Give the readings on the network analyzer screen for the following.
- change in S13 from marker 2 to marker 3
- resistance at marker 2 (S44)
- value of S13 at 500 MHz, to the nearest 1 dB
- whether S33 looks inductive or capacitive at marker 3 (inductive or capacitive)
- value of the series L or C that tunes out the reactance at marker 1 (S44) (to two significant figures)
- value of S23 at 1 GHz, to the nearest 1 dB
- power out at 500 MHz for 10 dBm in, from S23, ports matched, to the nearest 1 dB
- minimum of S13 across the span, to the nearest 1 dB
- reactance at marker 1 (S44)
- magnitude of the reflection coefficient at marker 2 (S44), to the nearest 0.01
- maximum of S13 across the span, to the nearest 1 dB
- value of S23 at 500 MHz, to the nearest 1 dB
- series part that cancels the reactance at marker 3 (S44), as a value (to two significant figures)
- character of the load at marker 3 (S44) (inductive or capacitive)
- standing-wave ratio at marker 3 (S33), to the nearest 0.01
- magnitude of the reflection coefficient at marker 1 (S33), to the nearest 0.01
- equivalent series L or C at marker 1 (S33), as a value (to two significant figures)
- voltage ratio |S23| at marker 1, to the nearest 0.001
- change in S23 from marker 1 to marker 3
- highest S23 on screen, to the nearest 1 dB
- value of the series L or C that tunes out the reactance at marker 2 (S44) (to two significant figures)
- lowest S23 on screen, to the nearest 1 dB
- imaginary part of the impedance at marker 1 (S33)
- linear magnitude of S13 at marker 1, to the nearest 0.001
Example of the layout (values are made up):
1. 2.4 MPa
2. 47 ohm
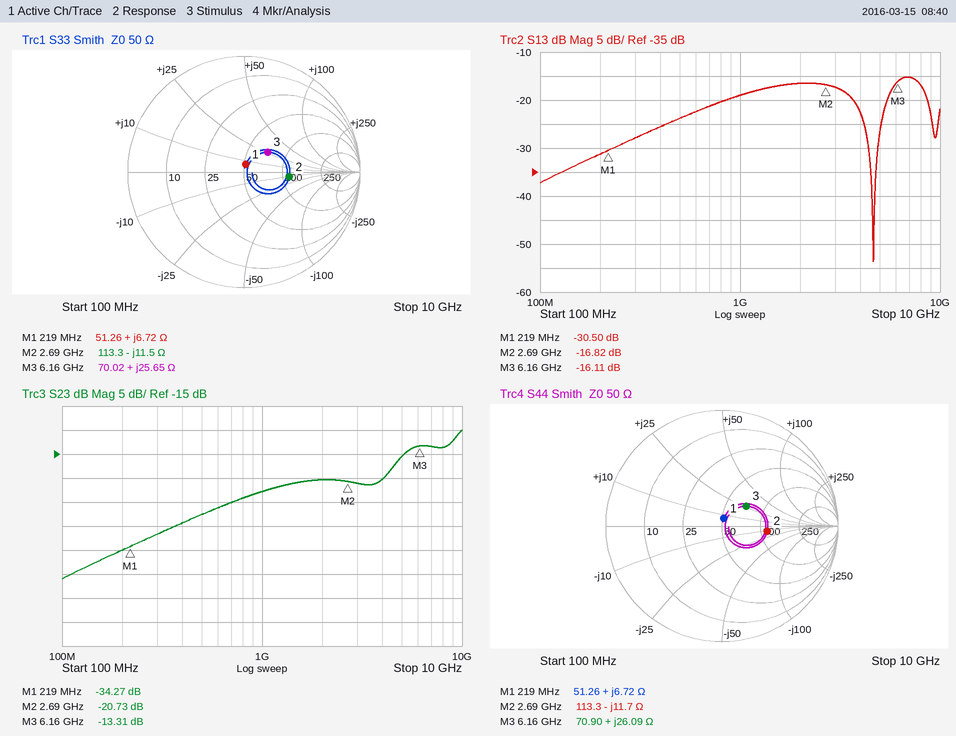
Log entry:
1. 0.71 dB
2. 113.3 Ω
3. -24 dB
4. inductive
5. 110 pF
6. -23 dB
7. -18 dBm
8. -54 dB
9. +6.72 Ω
10. 0.39
11. -15 dB
12. -28 dB
13. 990 fF
14. inductive
15. 1.72
16. 0.07
17. 4.9 nH
18. 0.019
19. 20.96 dB
20. -10 dB
21. 690 pH
22. -41 dB
23. +6.72 Ω
24. 0.030
